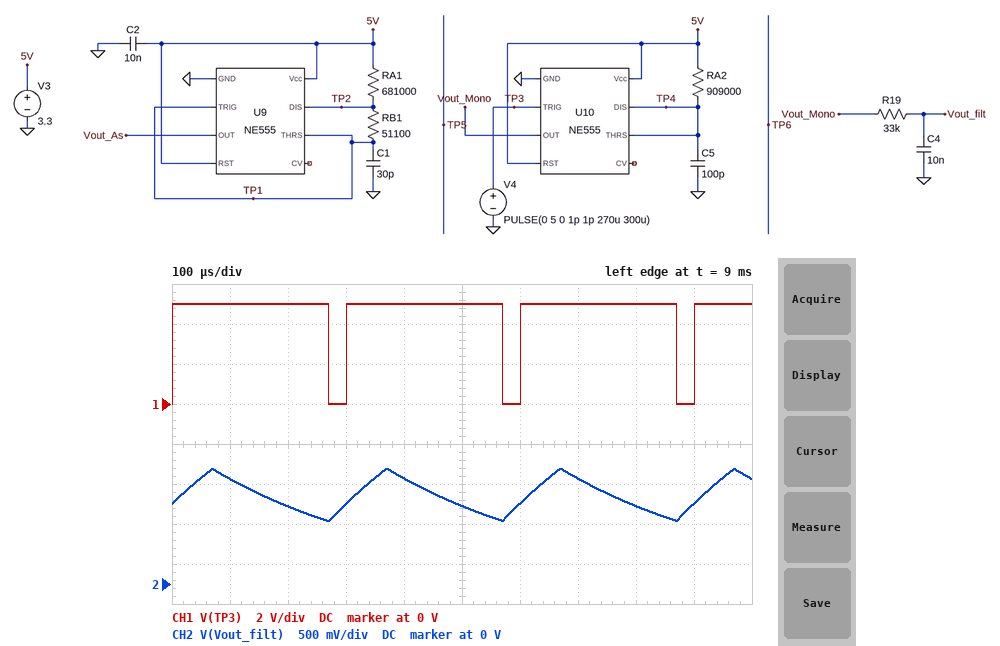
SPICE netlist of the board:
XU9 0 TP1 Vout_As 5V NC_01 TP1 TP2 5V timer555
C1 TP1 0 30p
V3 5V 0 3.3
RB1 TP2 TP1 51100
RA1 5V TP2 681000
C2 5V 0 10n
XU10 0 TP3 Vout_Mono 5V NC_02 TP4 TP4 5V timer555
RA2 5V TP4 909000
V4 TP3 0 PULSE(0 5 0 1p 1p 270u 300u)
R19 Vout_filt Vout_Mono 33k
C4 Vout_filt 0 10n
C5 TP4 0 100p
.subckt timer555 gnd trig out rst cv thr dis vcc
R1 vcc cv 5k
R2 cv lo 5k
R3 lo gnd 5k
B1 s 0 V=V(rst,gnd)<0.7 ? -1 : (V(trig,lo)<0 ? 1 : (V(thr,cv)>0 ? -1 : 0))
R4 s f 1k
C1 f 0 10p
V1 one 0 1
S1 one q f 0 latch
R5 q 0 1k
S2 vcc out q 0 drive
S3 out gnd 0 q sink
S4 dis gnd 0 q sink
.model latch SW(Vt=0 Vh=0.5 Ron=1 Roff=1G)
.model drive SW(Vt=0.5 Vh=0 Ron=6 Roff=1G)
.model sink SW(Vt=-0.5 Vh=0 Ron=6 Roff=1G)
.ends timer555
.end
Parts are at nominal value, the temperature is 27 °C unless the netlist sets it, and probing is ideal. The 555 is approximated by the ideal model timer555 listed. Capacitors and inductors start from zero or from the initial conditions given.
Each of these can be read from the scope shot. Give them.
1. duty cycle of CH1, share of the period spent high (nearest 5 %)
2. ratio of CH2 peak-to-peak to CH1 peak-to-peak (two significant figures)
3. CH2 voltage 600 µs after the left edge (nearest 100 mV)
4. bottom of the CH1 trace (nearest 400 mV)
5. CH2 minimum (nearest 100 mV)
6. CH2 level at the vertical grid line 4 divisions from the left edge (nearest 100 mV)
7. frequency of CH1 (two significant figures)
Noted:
90 %
0.13
1.0 V
0 V
800 mV
1.3 V
3.3 kHz
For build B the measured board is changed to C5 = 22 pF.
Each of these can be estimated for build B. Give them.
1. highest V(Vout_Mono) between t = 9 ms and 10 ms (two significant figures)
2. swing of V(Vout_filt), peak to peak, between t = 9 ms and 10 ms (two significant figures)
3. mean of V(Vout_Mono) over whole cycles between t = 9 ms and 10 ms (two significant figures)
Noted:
3.3 V
270 mV
330 mV
